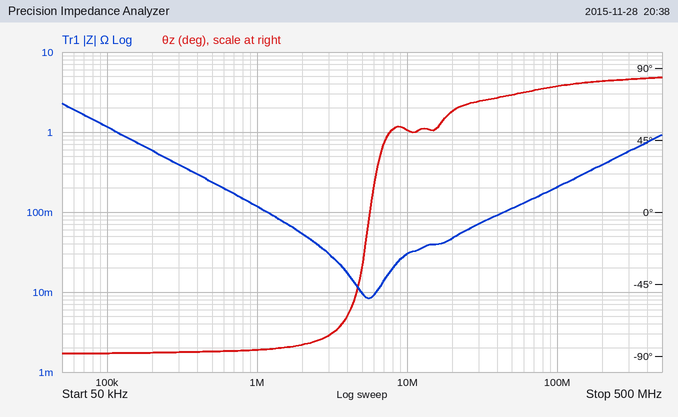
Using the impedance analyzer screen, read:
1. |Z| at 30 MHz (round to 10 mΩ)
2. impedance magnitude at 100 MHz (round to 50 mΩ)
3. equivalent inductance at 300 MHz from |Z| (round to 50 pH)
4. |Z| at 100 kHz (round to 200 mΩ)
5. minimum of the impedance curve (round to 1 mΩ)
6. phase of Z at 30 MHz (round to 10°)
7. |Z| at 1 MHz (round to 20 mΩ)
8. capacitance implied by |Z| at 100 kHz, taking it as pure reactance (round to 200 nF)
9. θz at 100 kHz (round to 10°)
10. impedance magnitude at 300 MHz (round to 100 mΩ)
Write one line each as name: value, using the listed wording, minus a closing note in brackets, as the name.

|Z| at 30 MHz: 70 mΩ
impedance magnitude at 100 MHz: 200 mΩ
equivalent inductance at 300 MHz from |Z|: 300 pH
|Z| at 100 kHz: 1.2 Ω
minimum of the impedance curve: 8 mΩ
phase of Z at 30 MHz: 70°
|Z| at 1 MHz: 120 mΩ
capacitance implied by |Z| at 100 kHz, taking it as pure reactance: 1.4 µF
θz at 100 kHz: -90°
impedance magnitude at 300 MHz: 600 mΩ
